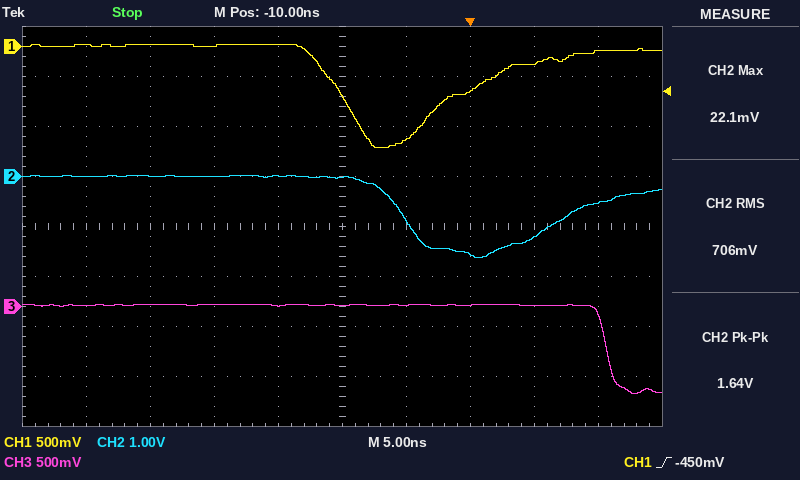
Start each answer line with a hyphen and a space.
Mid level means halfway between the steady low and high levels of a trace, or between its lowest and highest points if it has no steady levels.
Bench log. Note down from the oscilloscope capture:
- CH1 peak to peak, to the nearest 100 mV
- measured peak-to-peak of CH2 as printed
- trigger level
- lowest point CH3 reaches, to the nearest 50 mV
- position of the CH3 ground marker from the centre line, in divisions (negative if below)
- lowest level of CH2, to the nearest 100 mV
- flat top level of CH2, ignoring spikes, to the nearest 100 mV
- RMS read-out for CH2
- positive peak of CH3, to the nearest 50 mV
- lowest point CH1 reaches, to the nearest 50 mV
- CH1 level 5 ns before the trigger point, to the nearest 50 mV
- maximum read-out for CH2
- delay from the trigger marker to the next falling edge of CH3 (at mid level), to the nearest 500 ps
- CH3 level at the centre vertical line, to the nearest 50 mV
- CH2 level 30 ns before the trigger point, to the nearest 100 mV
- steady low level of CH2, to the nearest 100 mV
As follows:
- 1.00 V
- 1.64 V
- -450 mV
- -850 mV
- -1.6 div
- -1.6 V
- 0.0 V
- 706 mV
- 0 mV
- -1.00 V
- -950 mV
- 22.1 mV
- 10.5 ns
- 0 mV
- 0.0 V
- -1.4 V
